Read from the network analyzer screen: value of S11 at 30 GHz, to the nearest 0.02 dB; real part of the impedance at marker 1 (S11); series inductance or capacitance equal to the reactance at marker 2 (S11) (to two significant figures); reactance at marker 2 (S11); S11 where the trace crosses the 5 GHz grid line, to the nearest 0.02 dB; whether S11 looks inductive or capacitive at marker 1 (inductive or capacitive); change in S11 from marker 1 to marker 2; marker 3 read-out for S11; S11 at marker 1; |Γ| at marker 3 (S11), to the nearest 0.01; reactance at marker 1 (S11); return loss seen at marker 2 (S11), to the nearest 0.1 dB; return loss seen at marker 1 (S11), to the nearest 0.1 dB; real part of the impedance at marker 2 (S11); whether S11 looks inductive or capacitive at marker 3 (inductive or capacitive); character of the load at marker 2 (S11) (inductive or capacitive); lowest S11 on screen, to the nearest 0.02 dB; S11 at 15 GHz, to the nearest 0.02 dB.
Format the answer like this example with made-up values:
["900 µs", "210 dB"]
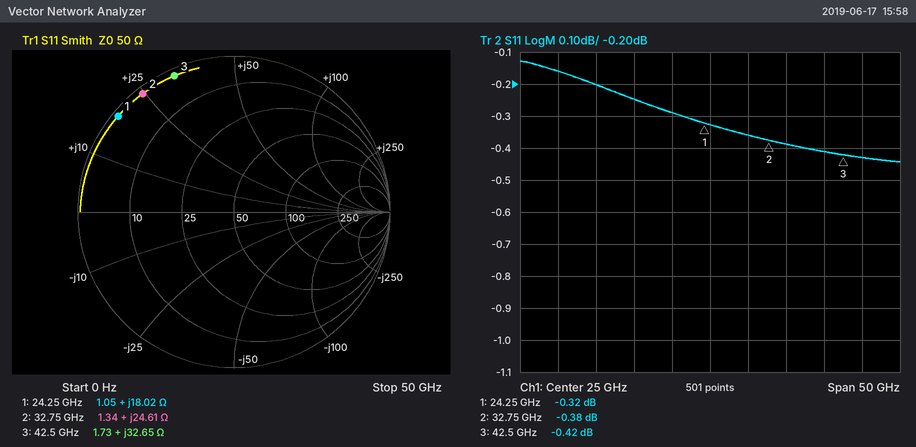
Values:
["-0.36 dB", "1.05 Ω", "120 pH", "+24.61 Ω", "-0.16 dB", "inductive", "-0.06 dB", "-0.42 dB", "-0.32 dB", "0.95", "+18.02 Ω", "0.4 dB", "0.3 dB", "1.34 Ω", "inductive", "inductive", "-0.44 dB", "-0.24 dB"]
